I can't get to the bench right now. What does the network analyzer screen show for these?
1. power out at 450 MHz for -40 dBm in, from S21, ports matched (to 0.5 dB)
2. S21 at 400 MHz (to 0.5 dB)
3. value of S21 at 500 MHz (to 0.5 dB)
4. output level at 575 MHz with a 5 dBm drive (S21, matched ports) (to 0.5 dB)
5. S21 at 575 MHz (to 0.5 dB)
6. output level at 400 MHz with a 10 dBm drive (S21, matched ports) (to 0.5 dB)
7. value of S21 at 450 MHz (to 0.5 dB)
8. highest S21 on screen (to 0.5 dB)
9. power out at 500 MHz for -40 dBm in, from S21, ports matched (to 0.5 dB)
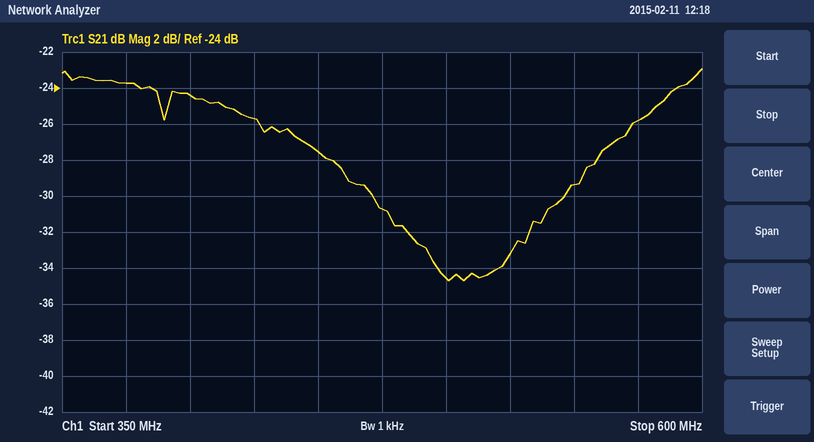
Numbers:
-67.5 dBm
-24.5 dB
-34.5 dB
-21.0 dBm
-26.0 dB
-14.5 dBm
-27.5 dB
-23.0 dB
-74.5 dBm
